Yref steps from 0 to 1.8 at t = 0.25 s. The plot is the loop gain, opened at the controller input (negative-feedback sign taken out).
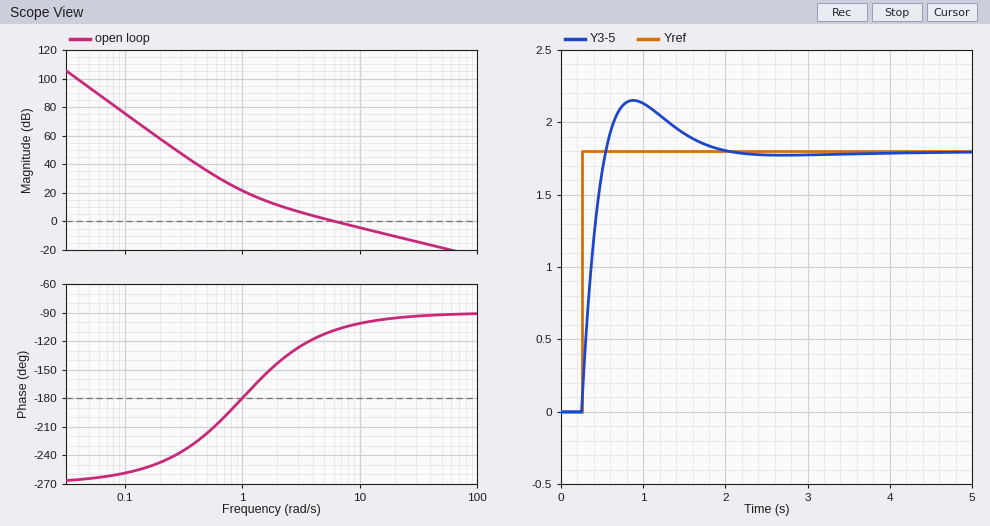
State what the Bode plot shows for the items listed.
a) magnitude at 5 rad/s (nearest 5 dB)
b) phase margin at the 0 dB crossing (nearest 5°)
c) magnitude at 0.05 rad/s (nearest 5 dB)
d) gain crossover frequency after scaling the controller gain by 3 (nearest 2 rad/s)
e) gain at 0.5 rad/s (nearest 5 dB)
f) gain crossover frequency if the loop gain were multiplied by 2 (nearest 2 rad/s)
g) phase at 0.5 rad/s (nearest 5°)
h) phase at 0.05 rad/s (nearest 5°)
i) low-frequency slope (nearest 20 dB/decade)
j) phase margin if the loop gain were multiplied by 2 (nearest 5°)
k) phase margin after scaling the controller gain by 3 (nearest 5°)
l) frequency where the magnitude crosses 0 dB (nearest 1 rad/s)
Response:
0 dB
70°
95 dB
18 rad/s
35 dB
12 rad/s
-215°
-265°
-60 dB/decade
80°
85°
6 rad/s
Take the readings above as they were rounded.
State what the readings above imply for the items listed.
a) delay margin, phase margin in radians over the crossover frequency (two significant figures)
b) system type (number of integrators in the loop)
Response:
0.20 s
3
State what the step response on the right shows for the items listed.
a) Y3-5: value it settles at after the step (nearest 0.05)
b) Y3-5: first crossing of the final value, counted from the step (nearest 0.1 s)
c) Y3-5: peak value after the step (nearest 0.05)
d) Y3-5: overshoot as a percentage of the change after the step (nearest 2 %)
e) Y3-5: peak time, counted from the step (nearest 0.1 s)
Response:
1.80
0.3 s
2.15
20 %
0.6 s
